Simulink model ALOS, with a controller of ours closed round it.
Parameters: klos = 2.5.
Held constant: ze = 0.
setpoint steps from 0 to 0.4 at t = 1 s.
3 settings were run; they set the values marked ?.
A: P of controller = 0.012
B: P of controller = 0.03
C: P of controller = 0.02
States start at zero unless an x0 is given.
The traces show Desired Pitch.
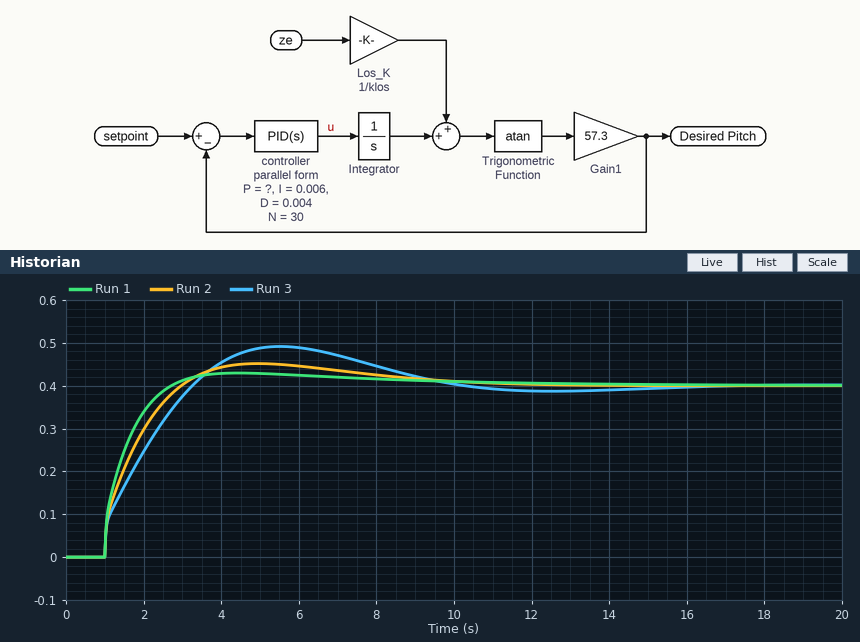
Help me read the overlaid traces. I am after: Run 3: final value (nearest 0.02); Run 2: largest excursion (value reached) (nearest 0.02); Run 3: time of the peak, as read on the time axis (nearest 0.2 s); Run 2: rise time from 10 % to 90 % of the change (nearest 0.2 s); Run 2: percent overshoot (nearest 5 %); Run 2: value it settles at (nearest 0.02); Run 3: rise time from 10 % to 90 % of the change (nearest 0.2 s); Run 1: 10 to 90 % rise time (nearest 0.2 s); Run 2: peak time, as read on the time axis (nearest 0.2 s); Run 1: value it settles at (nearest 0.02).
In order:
0.40
0.46
5.6 s
1.4 s
15 %
0.40
1.8 s
1.2 s
5.0 s
0.40
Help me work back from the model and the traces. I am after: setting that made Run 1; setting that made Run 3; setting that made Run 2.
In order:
B
A
C
